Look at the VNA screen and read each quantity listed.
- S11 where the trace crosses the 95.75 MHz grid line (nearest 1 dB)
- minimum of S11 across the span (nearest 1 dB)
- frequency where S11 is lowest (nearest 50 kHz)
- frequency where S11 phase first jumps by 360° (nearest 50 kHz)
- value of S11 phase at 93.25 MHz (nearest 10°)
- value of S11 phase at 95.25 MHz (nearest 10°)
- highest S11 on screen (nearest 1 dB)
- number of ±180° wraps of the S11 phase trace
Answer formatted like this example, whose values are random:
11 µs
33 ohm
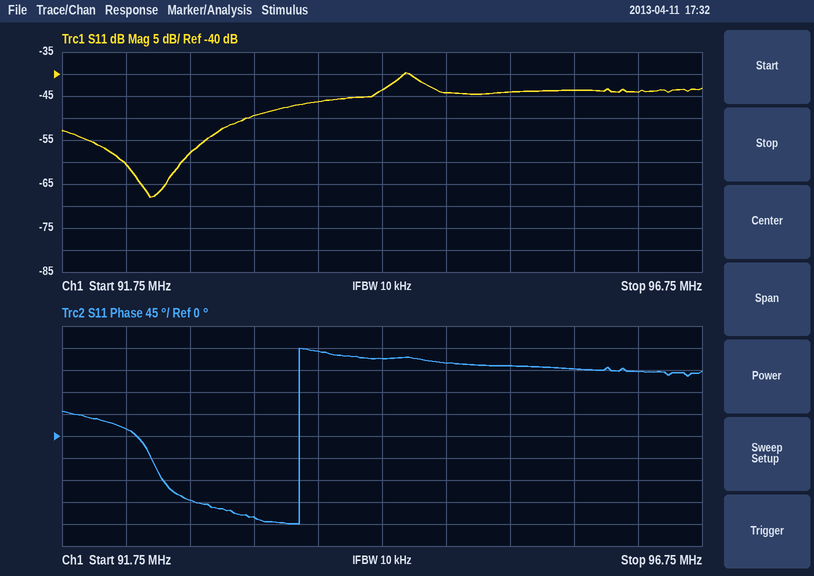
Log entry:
-44 dB
-68 dB
92.45 MHz
93.60 MHz
-170°
140°
-40 dB
1
